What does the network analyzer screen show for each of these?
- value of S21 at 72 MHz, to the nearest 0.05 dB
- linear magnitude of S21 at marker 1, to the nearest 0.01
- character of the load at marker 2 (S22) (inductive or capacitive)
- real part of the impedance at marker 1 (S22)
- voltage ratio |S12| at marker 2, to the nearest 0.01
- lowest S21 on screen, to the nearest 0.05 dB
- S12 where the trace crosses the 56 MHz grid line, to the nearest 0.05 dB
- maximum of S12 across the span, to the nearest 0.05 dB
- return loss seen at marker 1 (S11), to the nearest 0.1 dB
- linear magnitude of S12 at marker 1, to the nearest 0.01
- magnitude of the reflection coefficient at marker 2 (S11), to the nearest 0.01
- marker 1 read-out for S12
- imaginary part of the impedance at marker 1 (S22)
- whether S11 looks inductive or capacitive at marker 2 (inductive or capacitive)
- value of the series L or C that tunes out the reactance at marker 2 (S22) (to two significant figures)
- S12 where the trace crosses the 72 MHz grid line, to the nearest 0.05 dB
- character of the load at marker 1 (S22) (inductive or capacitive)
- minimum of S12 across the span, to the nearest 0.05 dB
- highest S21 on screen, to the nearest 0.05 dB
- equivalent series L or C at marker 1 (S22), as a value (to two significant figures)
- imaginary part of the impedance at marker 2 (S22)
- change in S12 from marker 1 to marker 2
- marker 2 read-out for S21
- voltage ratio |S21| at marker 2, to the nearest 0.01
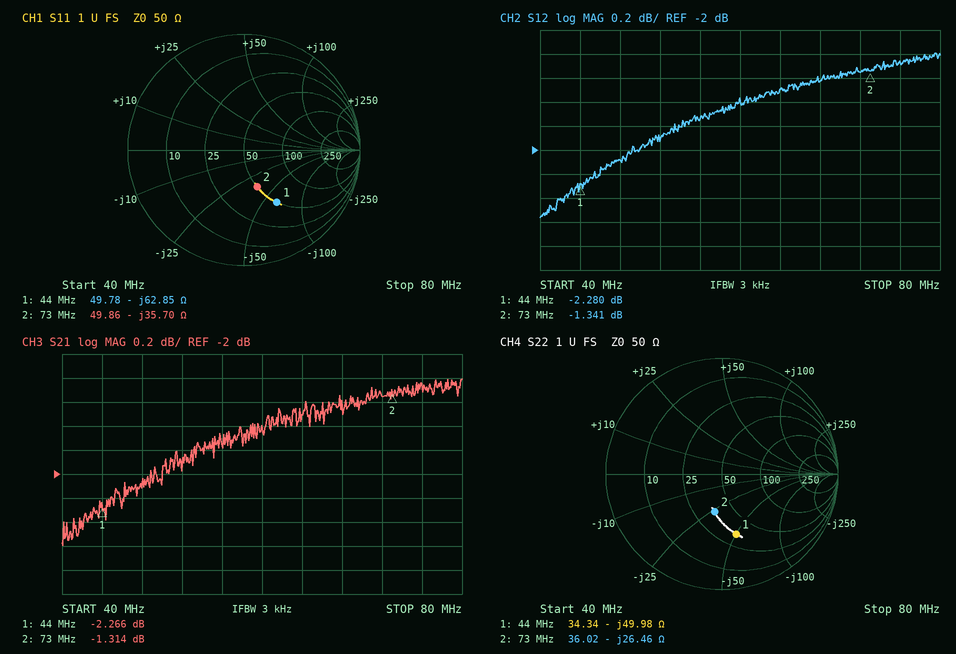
-1.35 dB
0.77
capacitive
34.34 Ω
0.86
-2.60 dB
-1.75 dB
-1.20 dB
5.5 dB
0.77
0.34
-2.280 dB
-49.98 Ω
capacitive
58 nH
-1.35 dB
capacitive
-2.55 dB
-1.20 dB
72 pF
-26.46 Ω
0.939 dB
-1.314 dB
0.86
